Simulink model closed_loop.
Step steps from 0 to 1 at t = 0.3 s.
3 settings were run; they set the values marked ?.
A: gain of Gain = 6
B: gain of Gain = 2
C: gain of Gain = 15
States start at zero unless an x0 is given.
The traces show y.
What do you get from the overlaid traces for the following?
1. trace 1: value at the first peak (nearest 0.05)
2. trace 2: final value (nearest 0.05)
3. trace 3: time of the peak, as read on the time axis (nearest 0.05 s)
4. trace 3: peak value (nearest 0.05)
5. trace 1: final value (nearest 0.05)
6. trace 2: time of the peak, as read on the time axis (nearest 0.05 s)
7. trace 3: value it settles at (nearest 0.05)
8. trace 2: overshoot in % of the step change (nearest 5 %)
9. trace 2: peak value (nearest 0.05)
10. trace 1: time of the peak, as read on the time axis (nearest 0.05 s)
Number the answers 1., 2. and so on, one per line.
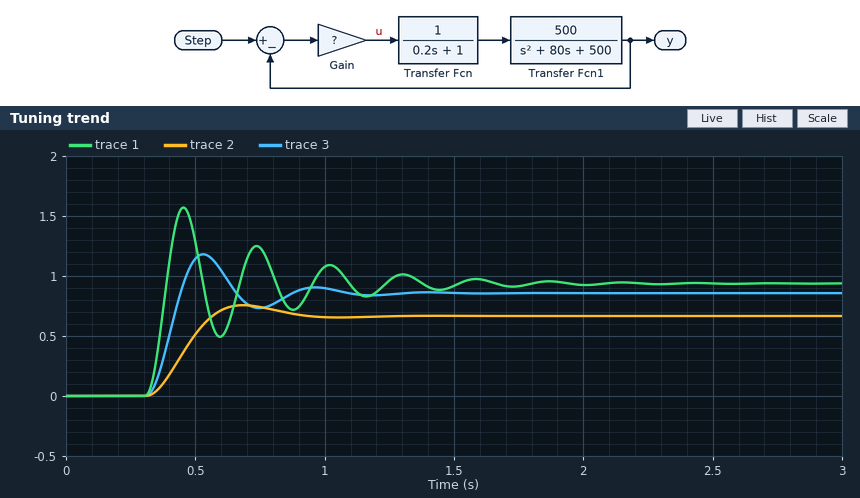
1. 1.55
2. 0.65
3. 0.55 s
4. 1.20
5. 0.95
6. 0.70 s
7. 0.85
8. 15 %
9. 0.75
10. 0.45 s
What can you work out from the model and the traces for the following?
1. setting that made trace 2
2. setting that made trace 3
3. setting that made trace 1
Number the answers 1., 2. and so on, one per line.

1. B
2. A
3. C
